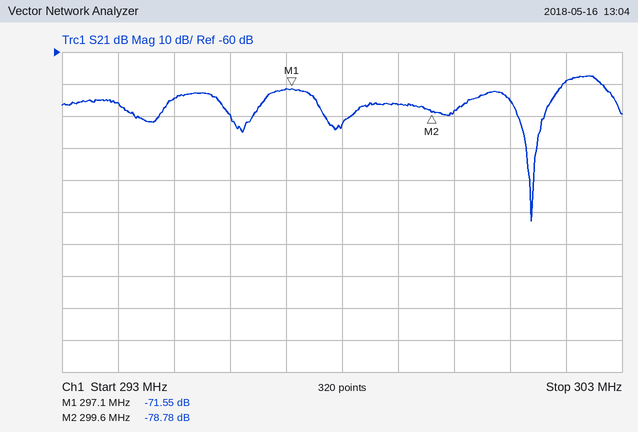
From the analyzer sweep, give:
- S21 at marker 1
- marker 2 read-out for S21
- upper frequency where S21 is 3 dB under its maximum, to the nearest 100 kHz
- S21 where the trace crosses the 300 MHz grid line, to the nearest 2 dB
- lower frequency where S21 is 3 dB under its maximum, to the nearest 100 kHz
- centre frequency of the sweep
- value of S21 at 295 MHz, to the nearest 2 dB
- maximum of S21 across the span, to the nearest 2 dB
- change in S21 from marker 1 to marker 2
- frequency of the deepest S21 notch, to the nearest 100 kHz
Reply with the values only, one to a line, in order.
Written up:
-71.55 dB
-78.78 dB
302.7 MHz
-78 dB
301.9 MHz
298 MHz
-74 dB
-68 dB
-7.23 dB
301.4 MHz
